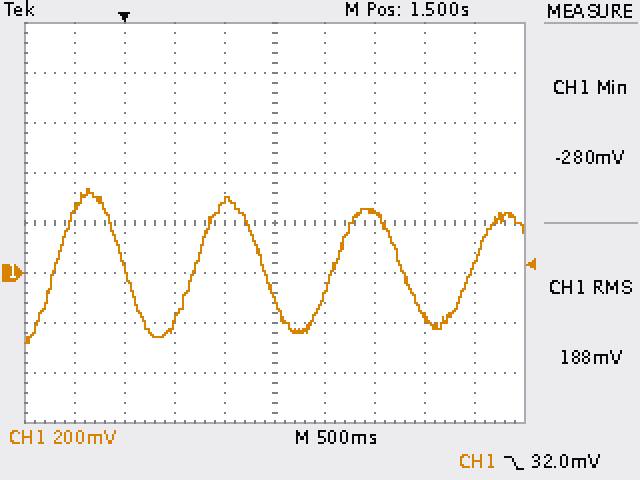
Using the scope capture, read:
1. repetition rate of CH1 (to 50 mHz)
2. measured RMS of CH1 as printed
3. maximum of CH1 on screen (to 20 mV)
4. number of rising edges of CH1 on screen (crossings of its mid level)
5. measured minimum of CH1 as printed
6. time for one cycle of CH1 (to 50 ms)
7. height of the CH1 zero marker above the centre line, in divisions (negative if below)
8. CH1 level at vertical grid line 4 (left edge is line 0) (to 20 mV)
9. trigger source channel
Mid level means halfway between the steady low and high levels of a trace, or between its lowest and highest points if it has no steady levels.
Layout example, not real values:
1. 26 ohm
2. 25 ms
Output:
1. 700 mHz
2. 188 mV
3. 340 mV
4. 4
5. -280 mV
6. 1.40 s
7. -1.0 div
8. 280 mV
9. CH1
